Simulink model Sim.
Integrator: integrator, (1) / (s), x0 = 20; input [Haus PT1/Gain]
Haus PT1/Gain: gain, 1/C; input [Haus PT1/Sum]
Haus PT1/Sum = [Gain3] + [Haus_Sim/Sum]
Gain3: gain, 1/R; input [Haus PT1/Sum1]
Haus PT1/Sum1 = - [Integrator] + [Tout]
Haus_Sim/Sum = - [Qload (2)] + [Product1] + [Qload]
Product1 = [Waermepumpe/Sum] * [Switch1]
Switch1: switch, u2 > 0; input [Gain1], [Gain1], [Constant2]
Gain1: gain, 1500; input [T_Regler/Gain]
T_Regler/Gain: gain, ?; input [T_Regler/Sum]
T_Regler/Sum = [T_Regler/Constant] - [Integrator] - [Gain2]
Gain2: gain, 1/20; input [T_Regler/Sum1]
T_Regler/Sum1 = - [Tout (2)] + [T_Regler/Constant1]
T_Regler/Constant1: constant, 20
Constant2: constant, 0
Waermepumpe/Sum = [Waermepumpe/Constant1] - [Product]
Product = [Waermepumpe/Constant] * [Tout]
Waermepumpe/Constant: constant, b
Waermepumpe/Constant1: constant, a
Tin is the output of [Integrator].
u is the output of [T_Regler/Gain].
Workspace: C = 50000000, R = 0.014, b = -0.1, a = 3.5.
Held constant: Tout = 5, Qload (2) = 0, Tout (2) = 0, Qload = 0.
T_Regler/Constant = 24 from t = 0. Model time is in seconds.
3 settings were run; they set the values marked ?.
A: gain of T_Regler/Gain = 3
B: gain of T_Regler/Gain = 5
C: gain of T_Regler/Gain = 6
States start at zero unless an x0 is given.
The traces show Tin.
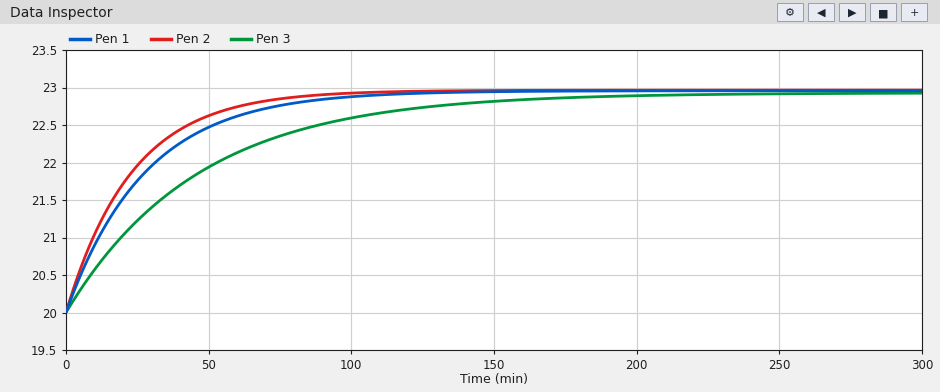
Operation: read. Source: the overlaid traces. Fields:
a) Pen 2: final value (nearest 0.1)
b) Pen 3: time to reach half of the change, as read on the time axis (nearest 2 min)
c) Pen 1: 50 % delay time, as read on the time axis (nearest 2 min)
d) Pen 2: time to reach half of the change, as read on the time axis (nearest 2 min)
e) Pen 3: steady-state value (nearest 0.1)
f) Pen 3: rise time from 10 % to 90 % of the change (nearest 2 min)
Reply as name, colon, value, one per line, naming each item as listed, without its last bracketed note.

Pen 2: final value: 23.0
Pen 3: time to reach half of the change, as read on the time axis: 32 min
Pen 1: 50 % delay time, as read on the time axis: 20 min
Pen 2: time to reach half of the change, as read on the time axis: 16 min
Pen 3: steady-state value: 22.9
Pen 3: rise time from 10 % to 90 % of the change: 102 min
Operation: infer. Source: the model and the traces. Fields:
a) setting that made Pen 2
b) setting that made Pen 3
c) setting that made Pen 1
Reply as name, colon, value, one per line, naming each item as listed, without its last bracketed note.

setting that made Pen 2: C
setting that made Pen 3: A
setting that made Pen 1: B
